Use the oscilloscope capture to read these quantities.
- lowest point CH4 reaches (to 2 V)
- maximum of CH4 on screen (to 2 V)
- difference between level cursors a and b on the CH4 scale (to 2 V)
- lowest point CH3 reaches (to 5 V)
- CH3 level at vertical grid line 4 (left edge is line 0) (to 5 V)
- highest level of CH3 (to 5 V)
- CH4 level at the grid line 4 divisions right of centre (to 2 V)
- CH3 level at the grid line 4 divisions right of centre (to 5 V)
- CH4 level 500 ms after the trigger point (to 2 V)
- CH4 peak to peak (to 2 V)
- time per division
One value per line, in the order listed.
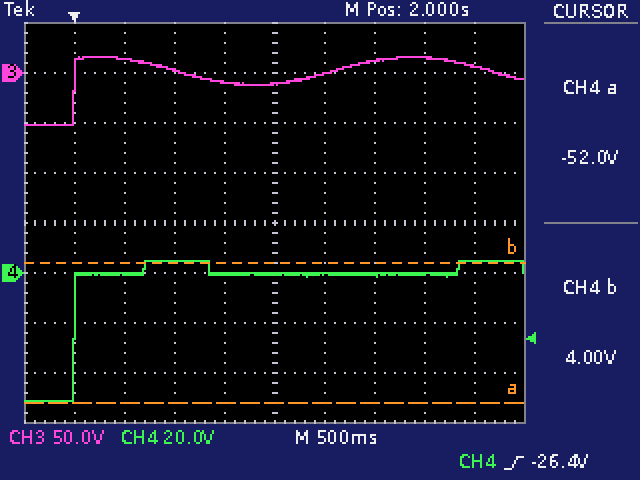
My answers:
-52 V
4 V
56 V
-50 V
-10 V
15 V
4 V
5 V
0 V
56 V
500 ms
